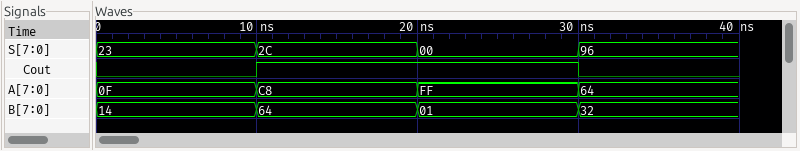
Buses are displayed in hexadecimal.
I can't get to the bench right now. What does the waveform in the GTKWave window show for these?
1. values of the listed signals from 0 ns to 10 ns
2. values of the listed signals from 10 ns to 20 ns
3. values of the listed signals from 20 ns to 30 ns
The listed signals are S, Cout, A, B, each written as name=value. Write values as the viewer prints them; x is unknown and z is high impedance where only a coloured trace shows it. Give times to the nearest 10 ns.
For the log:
S=23, Cout=0, A=0F, B=14
S=2C, Cout=1, A=C8, B=64
S=00, Cout=1, A=FF, B=01
